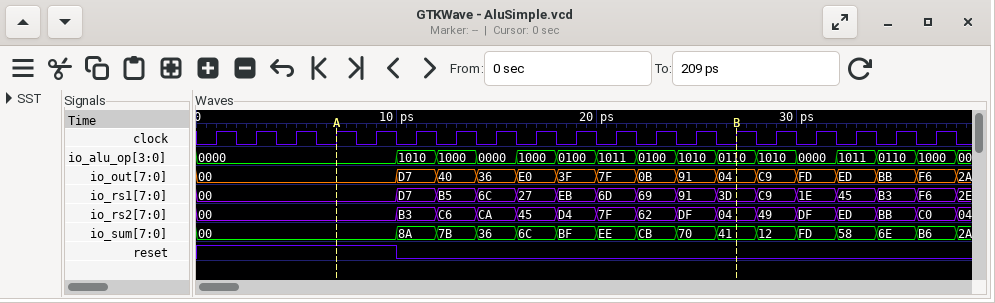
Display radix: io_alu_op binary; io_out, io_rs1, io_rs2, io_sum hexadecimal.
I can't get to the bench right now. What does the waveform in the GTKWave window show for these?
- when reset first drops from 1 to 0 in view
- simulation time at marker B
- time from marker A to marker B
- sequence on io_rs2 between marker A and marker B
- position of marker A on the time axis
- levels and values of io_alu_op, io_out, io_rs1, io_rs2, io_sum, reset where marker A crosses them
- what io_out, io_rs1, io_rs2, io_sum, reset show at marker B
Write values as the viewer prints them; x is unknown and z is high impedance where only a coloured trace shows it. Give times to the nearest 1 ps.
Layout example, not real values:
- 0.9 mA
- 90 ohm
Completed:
- 10 ps
- 27 ps
- 20 ps
- 00, B3, C6, CA, 45, D4, 7F, 62, DF, 04
- 7 ps
- io_alu_op=0000, io_out=00, io_rs1=00, io_rs2=00, io_sum=00, reset=1
- io_out=04, io_rs1=3D, io_rs2=04, io_sum=41, reset=0
